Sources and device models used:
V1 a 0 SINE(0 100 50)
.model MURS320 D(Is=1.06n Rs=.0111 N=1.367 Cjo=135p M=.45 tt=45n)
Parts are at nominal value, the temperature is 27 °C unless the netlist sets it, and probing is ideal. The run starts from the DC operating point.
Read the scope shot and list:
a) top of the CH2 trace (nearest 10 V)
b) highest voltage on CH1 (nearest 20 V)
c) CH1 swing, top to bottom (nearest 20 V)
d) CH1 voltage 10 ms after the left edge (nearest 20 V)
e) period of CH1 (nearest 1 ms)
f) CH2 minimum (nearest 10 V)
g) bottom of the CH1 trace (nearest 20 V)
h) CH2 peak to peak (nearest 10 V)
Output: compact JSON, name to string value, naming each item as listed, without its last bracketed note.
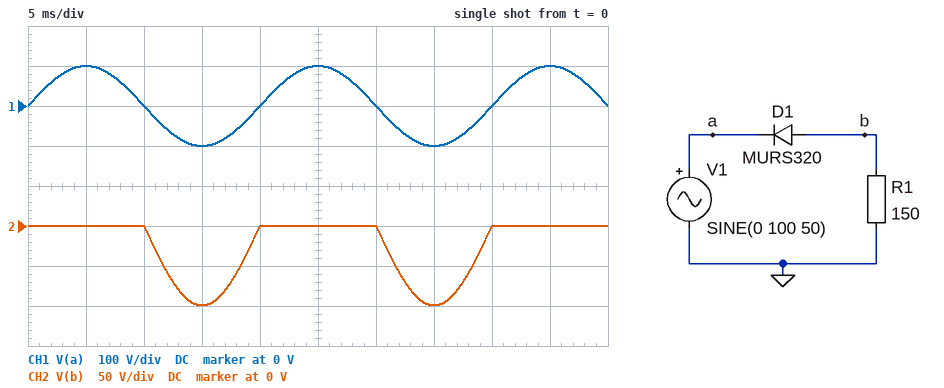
{"top of the CH2 trace": "0 V", "highest voltage on CH1": "100 V", "CH1 swing, top to bottom": "200 V", "CH1 voltage 10 ms after the left edge": "0 V", "period of CH1": "20 ms", "CH2 minimum": "-100 V", "bottom of the CH1 trace": "-100 V", "CH2 peak to peak": "100 V"}
